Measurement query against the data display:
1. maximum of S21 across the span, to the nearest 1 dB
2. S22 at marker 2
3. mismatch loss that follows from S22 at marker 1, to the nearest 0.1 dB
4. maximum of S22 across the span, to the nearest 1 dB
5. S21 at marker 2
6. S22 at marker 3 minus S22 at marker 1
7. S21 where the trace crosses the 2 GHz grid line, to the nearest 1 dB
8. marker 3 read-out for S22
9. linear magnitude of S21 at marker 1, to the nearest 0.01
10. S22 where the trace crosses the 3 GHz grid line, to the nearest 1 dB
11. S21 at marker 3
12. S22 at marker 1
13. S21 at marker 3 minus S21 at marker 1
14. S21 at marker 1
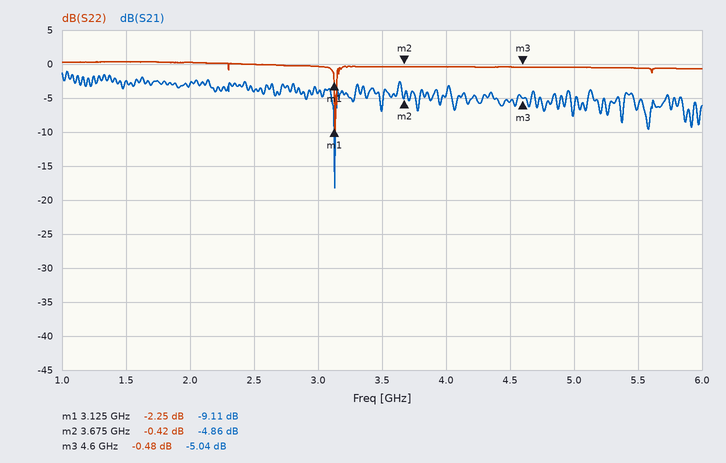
-1 dB
-0.42 dB
3.9 dB
0 dB
-4.86 dB
1.77 dB
-3 dB
-0.48 dB
0.35
0 dB
-5.04 dB
-2.25 dB
4.07 dB
-9.11 dB
